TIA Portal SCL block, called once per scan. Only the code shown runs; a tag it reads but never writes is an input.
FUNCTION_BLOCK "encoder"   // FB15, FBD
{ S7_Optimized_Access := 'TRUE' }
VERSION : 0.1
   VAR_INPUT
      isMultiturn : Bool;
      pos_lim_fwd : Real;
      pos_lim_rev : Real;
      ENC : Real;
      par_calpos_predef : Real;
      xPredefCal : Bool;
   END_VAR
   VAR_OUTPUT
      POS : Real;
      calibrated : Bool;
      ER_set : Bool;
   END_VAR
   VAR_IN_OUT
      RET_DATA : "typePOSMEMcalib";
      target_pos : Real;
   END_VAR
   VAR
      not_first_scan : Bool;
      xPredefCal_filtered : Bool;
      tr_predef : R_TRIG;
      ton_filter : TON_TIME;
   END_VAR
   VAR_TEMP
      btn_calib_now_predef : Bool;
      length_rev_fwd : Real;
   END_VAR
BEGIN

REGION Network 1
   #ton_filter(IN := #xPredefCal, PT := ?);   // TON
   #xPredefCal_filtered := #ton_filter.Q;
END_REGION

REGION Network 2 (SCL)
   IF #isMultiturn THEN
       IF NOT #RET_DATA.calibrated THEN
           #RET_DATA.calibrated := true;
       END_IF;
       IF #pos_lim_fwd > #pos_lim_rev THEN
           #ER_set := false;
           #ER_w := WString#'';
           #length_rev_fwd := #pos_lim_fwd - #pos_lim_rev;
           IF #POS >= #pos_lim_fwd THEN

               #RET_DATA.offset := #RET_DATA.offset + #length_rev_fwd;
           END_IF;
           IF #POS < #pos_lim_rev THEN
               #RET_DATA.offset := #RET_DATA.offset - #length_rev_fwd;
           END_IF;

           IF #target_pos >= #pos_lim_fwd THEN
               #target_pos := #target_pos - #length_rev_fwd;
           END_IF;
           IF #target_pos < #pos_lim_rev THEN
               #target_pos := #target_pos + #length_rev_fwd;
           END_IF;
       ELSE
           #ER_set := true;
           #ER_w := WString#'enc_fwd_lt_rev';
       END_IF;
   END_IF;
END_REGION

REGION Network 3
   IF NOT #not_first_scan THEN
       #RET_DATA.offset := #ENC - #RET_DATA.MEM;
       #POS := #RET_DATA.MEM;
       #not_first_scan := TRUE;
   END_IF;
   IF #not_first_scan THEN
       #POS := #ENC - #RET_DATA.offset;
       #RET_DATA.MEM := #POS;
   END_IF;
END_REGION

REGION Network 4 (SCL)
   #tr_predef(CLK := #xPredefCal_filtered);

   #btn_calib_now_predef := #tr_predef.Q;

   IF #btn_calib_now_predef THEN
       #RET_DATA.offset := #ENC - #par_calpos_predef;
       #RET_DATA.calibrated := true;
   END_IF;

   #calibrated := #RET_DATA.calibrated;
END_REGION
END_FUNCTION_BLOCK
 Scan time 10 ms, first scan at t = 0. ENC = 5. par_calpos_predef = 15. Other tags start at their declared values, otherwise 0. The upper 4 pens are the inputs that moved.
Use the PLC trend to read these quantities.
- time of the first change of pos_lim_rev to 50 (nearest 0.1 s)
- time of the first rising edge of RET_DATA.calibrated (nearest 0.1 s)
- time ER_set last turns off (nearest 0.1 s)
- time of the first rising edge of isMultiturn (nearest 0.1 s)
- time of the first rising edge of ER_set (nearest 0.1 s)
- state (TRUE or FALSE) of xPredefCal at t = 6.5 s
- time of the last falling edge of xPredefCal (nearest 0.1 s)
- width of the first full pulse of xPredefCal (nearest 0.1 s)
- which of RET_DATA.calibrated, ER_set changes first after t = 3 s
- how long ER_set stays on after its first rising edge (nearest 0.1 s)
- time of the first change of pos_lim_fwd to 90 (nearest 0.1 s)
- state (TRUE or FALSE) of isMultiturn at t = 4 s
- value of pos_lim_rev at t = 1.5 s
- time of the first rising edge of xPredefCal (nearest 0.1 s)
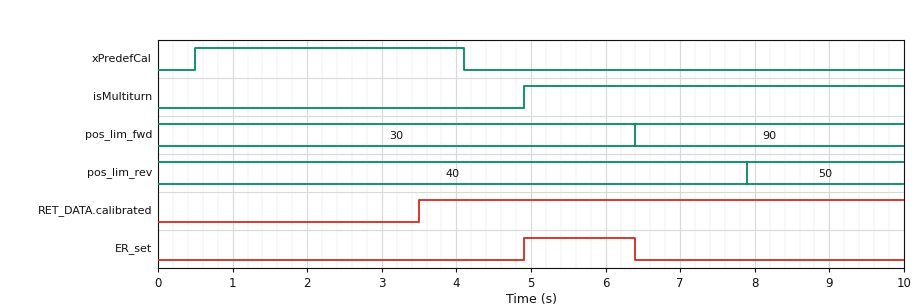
7.9 s
3.5 s
6.4 s
4.9 s
4.9 s
FALSE
4.1 s
3.6 s
RET_DATA.calibrated
1.5 s
6.4 s
FALSE
40
0.5 s
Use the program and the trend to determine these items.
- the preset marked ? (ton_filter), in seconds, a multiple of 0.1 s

3.0 s
